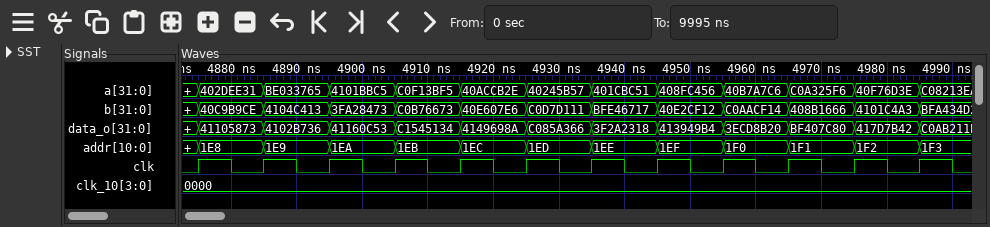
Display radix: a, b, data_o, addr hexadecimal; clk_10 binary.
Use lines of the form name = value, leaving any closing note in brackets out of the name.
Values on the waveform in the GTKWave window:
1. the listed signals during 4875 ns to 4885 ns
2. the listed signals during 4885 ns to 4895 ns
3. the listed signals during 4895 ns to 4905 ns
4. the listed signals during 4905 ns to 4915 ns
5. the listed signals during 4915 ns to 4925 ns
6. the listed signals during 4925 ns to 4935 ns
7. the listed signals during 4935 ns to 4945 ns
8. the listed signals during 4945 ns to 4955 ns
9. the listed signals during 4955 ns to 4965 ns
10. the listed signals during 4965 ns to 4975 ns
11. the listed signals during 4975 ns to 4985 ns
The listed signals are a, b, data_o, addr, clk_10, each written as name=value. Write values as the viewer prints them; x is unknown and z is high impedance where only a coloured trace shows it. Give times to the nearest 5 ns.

the listed signals during 4875 ns to 4885 ns = a=402DEE31, b=40C9B9CE, data_o=41105873, addr=1E8, clk_10=0000
the listed signals during 4885 ns to 4895 ns = a=BE033765, b=4104C413, data_o=4102B736, addr=1E9, clk_10=0000
the listed signals during 4895 ns to 4905 ns = a=4101BBC5, b=3FA28473, data_o=41160C53, addr=1EA, clk_10=0000
the listed signals during 4905 ns to 4915 ns = a=C0F13BF5, b=C0B76673, data_o=C1545134, addr=1EB, clk_10=0000
the listed signals during 4915 ns to 4925 ns = a=40ACCB2E, b=40E607E6, data_o=4149698A, addr=1EC, clk_10=0000
the listed signals during 4925 ns to 4935 ns = a=40245B57, b=C0D7D111, data_o=C085A366, addr=1ED, clk_10=0000
the listed signals during 4935 ns to 4945 ns = a=401CBC51, b=BFE46717, data_o=3F2A2318, addr=1EE, clk_10=0000
the listed signals during 4945 ns to 4955 ns = a=408FC456, b=40E2CF12, data_o=413949B4, addr=1EF, clk_10=0000
the listed signals during 4955 ns to 4965 ns = a=40B7A7C6, b=C0AACF14, data_o=3ECD8B20, addr=1F0, clk_10=0000
the listed signals during 4965 ns to 4975 ns = a=C0A325F6, b=408B1666, data_o=BF407C80, addr=1F1, clk_10=0000
the listed signals during 4975 ns to 4985 ns = a=40F76D3E, b=4101C4A3, data_o=417D7B42, addr=1F2, clk_10=0000
